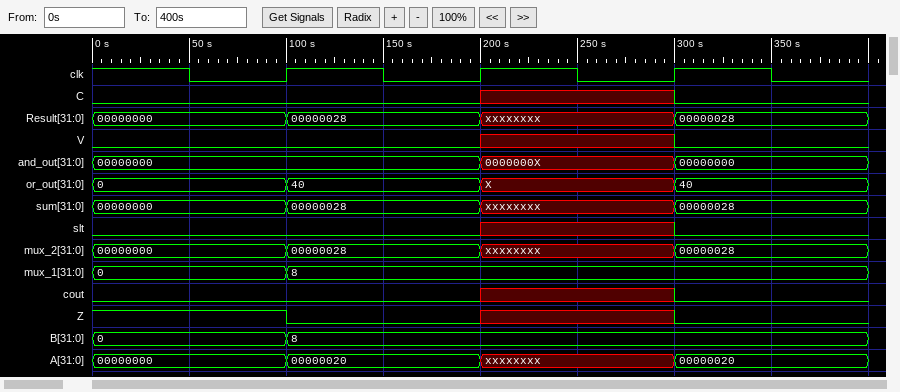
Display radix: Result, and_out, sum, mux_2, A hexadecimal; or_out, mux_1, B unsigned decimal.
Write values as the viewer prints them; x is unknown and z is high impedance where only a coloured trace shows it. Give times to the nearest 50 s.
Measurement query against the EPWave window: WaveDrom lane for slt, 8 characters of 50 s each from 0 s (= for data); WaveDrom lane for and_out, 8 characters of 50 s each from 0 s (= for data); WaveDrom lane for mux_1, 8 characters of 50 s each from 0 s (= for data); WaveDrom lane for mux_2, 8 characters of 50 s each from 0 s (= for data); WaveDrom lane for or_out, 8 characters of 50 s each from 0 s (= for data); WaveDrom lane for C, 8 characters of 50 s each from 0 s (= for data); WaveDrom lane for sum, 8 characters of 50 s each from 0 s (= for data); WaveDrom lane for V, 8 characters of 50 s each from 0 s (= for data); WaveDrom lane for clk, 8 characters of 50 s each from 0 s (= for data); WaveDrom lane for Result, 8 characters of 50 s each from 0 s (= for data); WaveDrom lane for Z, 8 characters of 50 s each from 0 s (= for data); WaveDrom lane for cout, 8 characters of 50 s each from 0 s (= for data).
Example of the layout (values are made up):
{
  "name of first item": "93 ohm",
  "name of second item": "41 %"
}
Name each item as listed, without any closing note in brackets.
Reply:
{
  "WaveDrom lane for slt, 8 characters of 50 s each from 0 s": "{name: 'slt', wave: '0...x.0.'}",
  "WaveDrom lane for and_out, 8 characters of 50 s each from 0 s": "{name: 'and_out', wave: '=...=.=.', data: '00000000 0000000X 00000000'}",
  "WaveDrom lane for mux_1, 8 characters of 50 s each from 0 s": "{name: 'mux_1', wave: '=.=.....', data: '0 8'}",
  "WaveDrom lane for mux_2, 8 characters of 50 s each from 0 s": "{name: 'mux_2', wave: '=.=.x.=.', data: '00000000 00000028 00000028'}",
  "WaveDrom lane for or_out, 8 characters of 50 s each from 0 s": "{name: 'or_out', wave: '=.=.=.=.', data: '0 40 X 40'}",
  "WaveDrom lane for C, 8 characters of 50 s each from 0 s": "{name: 'C', wave: '0...x.0.'}",
  "WaveDrom lane for sum, 8 characters of 50 s each from 0 s": "{name: 'sum', wave: '=.=.x.=.', data: '00000000 00000028 00000028'}",
  "WaveDrom lane for V, 8 characters of 50 s each from 0 s": "{name: 'V', wave: '0...x.0.'}",
  "WaveDrom lane for clk, 8 characters of 50 s each from 0 s": "{name: 'clk', wave: '10101010'}",
  "WaveDrom lane for Result, 8 characters of 50 s each from 0 s": "{name: 'Result', wave: '=.=.x.=.', data: '00000000 00000028 00000028'}",
  "WaveDrom lane for Z, 8 characters of 50 s each from 0 s": "{name: 'Z', wave: '1.0.x.0.'}",
  "WaveDrom lane for cout, 8 characters of 50 s each from 0 s": "{name: 'cout', wave: '0...x.0.'}"
}
